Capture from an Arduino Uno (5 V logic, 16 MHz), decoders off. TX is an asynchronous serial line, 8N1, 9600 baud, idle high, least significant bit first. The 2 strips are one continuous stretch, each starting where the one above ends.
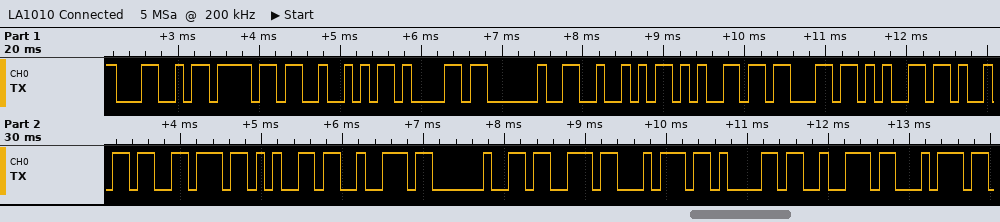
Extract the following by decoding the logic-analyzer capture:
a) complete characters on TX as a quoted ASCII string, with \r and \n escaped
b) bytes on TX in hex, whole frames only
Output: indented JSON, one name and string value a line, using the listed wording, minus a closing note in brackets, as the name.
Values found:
{
  "complete characters on TX as a quoted ASCII string, with \\r and \\n escaped": "\"LoRa Receiver start\"",
  "bytes on TX in hex, whole frames only": "4C 6F 52 61 20 52 65 63 65 69 76 65 72 20 73 74 61 72 74"
}
